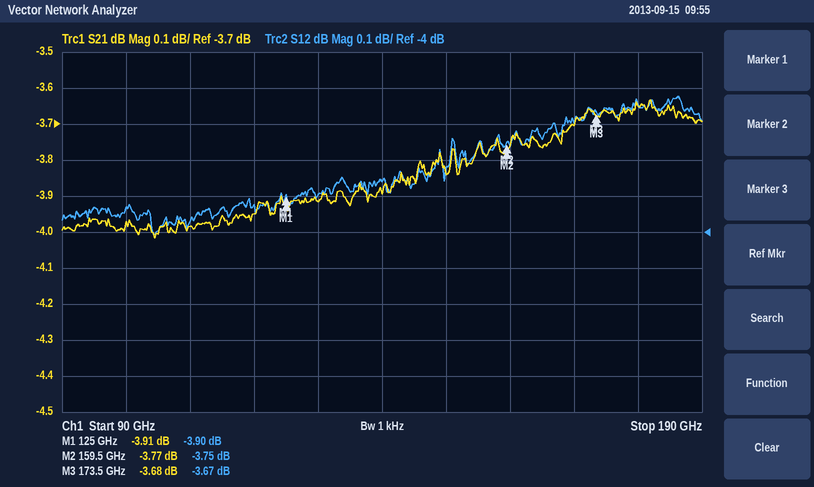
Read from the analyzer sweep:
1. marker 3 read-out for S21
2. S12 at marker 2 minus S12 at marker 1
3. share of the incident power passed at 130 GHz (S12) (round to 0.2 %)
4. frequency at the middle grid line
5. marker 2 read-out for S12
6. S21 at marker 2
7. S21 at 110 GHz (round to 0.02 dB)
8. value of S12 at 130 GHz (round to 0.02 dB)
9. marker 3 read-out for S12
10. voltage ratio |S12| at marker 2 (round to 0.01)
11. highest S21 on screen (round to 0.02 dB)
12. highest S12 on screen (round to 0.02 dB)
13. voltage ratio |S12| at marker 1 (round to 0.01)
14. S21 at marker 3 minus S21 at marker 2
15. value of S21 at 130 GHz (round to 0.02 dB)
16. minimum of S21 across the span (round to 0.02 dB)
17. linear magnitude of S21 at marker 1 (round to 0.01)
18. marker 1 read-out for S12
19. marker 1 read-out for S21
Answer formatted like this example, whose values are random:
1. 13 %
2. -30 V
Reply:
1. -3.68 dB
2. 0.15 dB
3. 40.8 %
4. 140 GHz
5. -3.75 dB
6. -3.77 dB
7. -3.98 dB
8. -3.90 dB
9. -3.67 dB
10. 0.65
11. -3.64 dB
12. -3.62 dB
13. 0.64
14. 0.09 dB
15. -3.92 dB
16. -4.02 dB
17. 0.64
18. -3.90 dB
19. -3.91 dB
